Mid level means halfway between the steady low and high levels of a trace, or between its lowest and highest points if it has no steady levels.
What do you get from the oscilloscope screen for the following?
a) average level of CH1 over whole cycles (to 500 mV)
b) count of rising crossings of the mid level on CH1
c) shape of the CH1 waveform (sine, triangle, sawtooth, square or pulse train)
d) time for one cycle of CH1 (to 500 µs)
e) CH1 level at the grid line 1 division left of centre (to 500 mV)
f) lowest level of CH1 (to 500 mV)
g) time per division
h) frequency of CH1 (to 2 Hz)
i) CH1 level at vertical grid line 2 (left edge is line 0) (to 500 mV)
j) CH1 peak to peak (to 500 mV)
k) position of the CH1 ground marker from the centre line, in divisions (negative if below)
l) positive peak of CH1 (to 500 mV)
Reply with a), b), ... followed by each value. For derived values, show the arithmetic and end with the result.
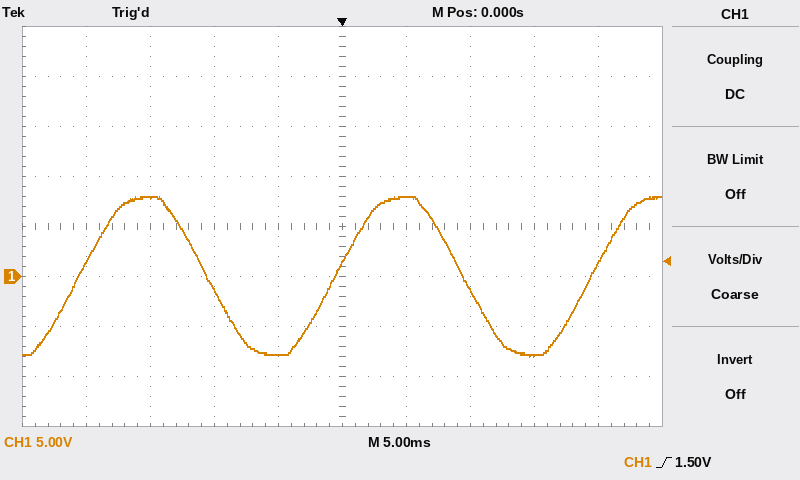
a) (8.0 V + (-8.0 V)) / 2 ≈ 0.0 V
b) 3
c) sine
d) 20.0 ms
e) -8.0 V
f) -8.0 V
g) 5 ms
h) 1 / 20.0 ms ≈ 50 Hz
i) 8.0 V
j) 8.0 V − (-8.0 V) = 16.0 V
k) -1.0 div
l) 8.0 V
